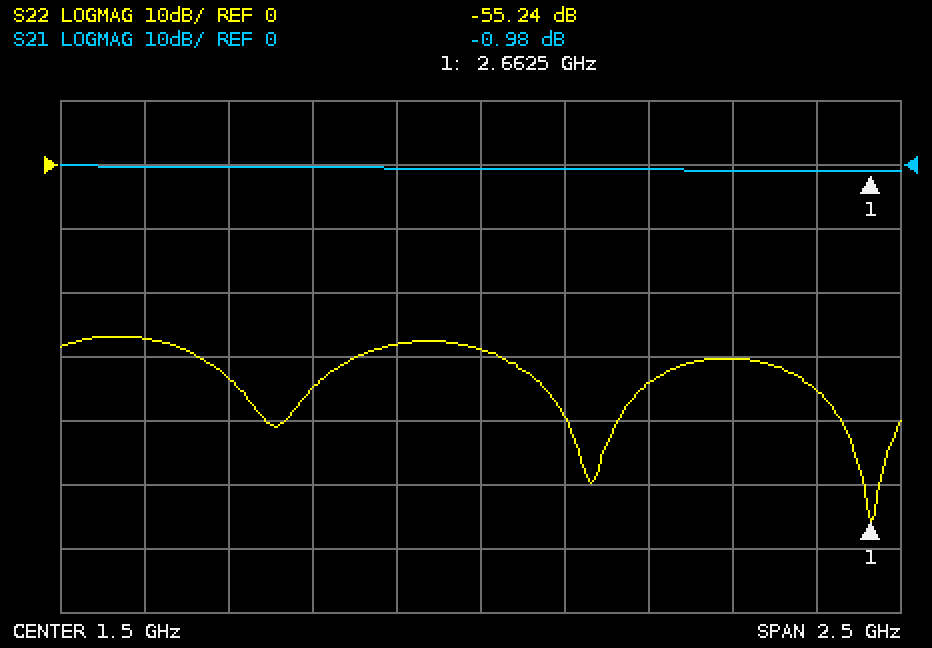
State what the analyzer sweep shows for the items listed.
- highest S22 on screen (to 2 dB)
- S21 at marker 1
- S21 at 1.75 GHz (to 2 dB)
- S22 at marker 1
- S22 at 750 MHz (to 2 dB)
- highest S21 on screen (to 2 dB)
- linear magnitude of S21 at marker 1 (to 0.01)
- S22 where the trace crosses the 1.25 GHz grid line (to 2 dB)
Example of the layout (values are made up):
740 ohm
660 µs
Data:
-26 dB
-0.98 dB
0 dB
-55.24 dB
-34 dB
0 dB
0.89
-28 dB
